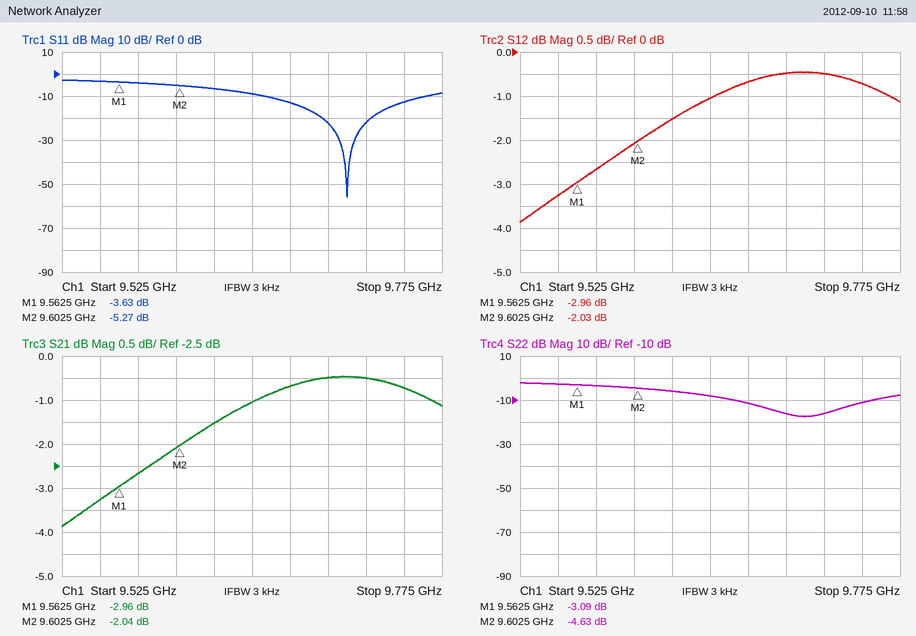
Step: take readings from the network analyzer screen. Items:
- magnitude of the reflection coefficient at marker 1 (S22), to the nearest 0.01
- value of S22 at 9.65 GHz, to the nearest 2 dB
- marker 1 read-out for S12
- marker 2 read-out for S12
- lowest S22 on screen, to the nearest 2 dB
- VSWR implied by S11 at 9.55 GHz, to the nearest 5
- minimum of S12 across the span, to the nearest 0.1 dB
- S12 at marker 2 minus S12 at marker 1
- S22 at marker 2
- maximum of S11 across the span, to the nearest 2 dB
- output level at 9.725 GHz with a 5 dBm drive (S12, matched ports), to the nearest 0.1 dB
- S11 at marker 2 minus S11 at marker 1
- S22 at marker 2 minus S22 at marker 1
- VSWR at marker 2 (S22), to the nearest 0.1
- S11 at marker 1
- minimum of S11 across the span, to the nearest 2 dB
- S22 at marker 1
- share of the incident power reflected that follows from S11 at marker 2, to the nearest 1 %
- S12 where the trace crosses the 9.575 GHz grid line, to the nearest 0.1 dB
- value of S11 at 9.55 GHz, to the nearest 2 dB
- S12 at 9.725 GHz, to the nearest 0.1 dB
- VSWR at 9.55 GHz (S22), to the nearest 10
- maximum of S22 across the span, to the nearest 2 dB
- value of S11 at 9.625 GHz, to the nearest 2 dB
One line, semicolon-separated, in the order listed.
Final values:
0.70; -8 dB; -2.96 dB; -2.03 dB; -18 dB; 5; -3.9 dB; 0.93 dB; -4.63 dB; -2 dB; 4.5 dBm; -1.64 dB; -1.54 dB; 3.8; -3.63 dB; -56 dB; -3.09 dB; 30 %; -2.7 dB; -4 dB; -0.5 dB; 10; -2 dB; -6 dB
